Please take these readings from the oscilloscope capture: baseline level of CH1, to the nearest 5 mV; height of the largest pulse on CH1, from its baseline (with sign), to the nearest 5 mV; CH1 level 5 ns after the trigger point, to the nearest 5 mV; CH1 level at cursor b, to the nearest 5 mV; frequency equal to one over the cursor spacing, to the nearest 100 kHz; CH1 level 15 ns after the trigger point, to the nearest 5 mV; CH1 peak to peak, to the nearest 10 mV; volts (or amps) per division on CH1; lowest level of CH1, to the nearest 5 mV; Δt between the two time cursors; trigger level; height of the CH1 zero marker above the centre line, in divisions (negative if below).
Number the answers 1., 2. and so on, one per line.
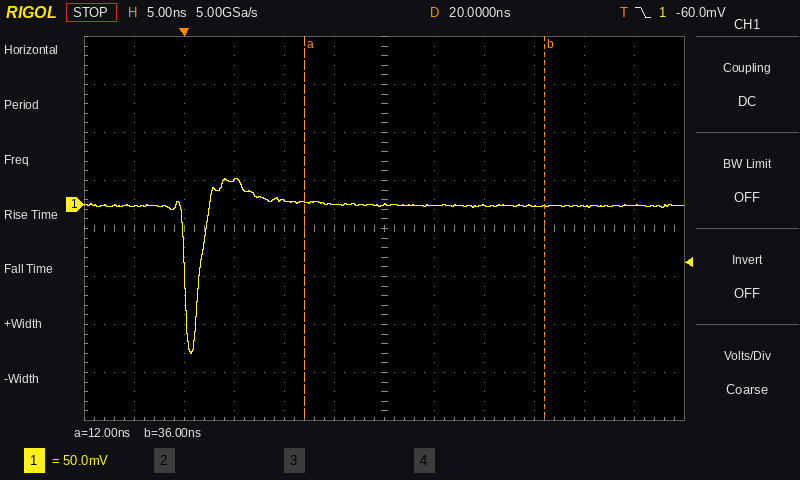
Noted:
1. 0 mV
2. -155 mV
3. 25 mV
4. 0 mV
5. 41.7 MHz
6. 0 mV
7. 180 mV
8. 50 mV
9. -155 mV
10. 24.0 ns
11. -60.0 mV
12. +0.5 div
